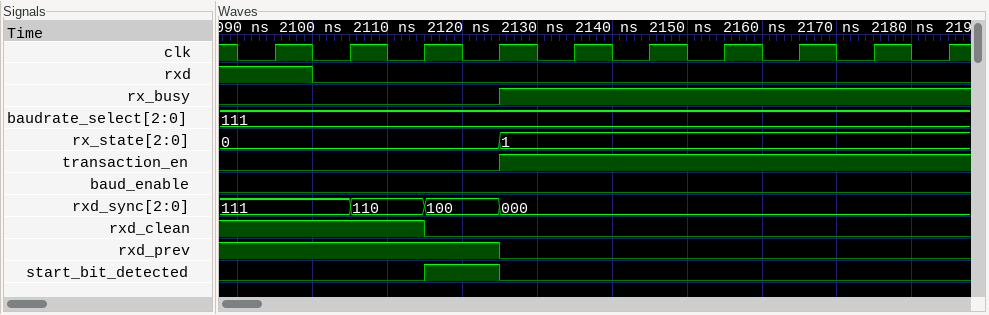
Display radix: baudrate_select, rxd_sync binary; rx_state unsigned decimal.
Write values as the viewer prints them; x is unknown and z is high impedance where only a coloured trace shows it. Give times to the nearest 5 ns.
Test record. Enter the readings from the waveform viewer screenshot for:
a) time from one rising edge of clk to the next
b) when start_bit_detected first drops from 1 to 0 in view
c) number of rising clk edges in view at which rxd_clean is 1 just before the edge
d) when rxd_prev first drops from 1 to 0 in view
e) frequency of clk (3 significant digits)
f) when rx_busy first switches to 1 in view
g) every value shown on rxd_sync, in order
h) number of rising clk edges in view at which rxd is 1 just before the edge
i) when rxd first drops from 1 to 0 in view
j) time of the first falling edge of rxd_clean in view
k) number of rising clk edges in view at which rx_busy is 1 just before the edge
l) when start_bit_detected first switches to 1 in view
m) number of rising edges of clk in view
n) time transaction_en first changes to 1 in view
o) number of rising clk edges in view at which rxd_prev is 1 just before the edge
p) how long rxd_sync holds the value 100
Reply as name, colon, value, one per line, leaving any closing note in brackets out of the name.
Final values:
time from one rising edge of clk to the next: 10 ns
when start_bit_detected first drops from 1 to 0 in view: 2125 ns
number of rising clk edges in view at which rxd_clean is 1 just before the edge: 3
when rxd_prev first drops from 1 to 0 in view: 2125 ns
frequency of clk: 100 MHz
when rx_busy first switches to 1 in view: 2125 ns
every value shown on rxd_sync, in order: 111, 110, 100, 000
number of rising clk edges in view at which rxd is 1 just before the edge: 1
when rxd first drops from 1 to 0 in view: 2100 ns
time of the first falling edge of rxd_clean in view: 2115 ns
number of rising clk edges in view at which rx_busy is 1 just before the edge: 6
when start_bit_detected first switches to 1 in view: 2115 ns
number of rising edges of clk in view: 10
time transaction_en first changes to 1 in view: 2125 ns
number of rising clk edges in view at which rxd_prev is 1 just before the edge: 4
how long rxd_sync holds the value 100: 10 ns
